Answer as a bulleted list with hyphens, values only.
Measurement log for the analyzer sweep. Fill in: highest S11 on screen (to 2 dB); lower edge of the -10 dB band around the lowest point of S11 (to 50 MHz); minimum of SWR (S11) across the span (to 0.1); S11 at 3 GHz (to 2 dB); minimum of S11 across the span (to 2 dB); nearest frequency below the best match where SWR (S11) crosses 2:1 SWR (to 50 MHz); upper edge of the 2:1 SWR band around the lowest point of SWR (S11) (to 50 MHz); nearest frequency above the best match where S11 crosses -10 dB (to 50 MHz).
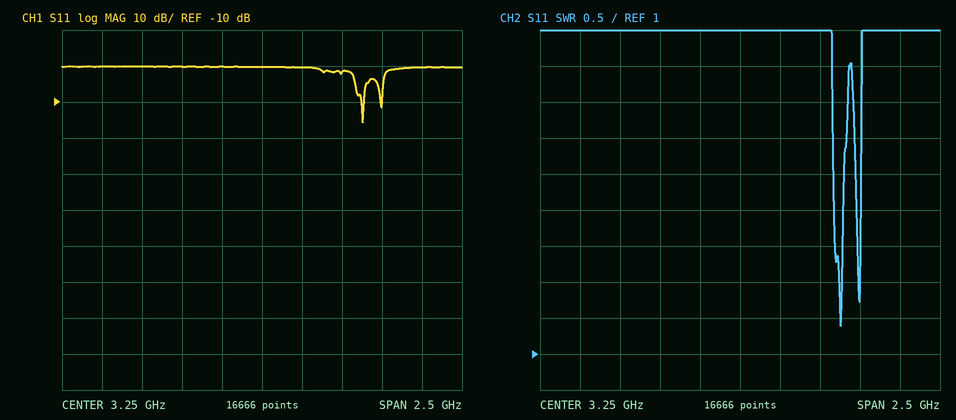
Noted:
- 0 dB
- 3.85 GHz
- 1.4
- 0 dB
- -16 dB
- 3.85 GHz
- 3.90 GHz
- 3.90 GHz
